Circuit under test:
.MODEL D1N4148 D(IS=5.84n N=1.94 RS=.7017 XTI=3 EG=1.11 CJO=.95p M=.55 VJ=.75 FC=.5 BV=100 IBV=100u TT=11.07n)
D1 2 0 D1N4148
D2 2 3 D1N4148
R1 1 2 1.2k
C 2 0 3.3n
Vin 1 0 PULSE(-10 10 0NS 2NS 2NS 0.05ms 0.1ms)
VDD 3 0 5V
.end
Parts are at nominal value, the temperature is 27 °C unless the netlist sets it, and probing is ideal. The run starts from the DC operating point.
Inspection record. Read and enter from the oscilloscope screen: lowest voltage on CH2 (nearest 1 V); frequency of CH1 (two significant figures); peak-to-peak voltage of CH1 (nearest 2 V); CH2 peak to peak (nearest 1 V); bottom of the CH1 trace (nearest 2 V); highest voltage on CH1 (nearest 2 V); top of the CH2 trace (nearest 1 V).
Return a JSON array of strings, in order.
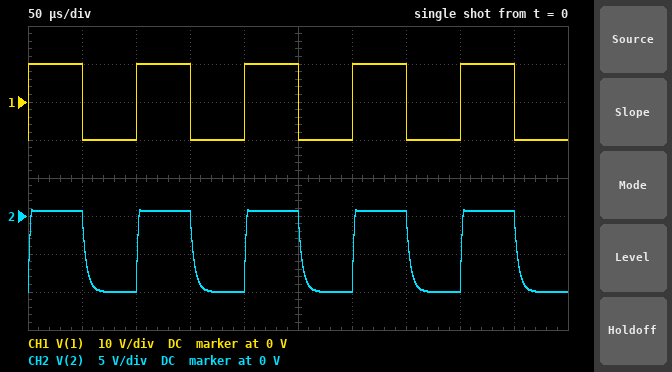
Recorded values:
["-10 V", "10 kHz", "20 V", "11 V", "-10 V", "10 V", "1 V"]
